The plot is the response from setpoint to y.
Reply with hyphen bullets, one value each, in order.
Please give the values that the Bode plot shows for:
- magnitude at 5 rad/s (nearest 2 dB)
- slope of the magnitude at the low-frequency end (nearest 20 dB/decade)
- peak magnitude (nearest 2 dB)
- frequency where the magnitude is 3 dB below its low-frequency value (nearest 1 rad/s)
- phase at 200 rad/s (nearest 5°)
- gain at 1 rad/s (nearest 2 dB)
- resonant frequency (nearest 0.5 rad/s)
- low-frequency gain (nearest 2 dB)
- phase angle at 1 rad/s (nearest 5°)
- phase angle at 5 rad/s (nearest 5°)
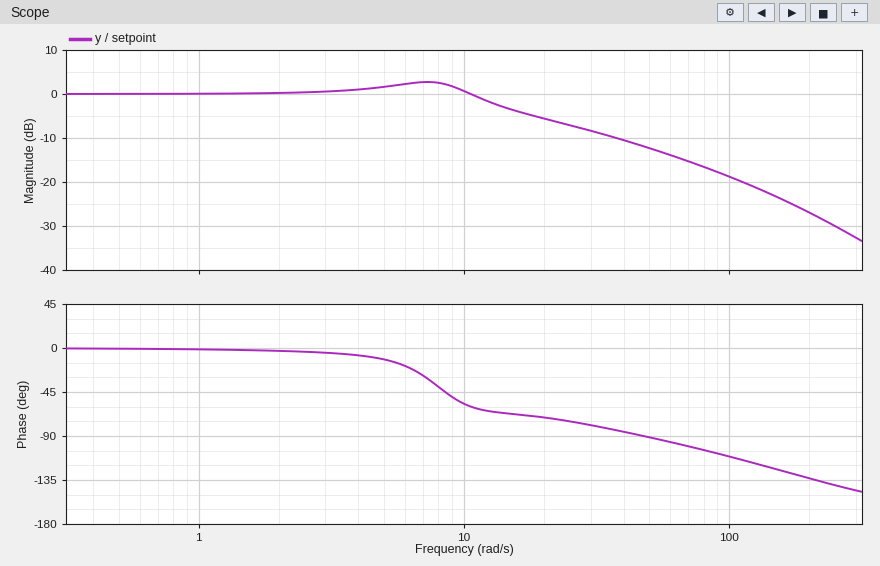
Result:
- 2 dB
- 0 dB/decade
- 2 dB
- 14 rad/s
- -135°
- 0 dB
- 7.0 rad/s
- 0 dB
- 0°
- -10°
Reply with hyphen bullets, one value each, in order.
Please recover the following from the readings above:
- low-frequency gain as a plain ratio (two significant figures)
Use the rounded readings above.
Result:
- 1.0
